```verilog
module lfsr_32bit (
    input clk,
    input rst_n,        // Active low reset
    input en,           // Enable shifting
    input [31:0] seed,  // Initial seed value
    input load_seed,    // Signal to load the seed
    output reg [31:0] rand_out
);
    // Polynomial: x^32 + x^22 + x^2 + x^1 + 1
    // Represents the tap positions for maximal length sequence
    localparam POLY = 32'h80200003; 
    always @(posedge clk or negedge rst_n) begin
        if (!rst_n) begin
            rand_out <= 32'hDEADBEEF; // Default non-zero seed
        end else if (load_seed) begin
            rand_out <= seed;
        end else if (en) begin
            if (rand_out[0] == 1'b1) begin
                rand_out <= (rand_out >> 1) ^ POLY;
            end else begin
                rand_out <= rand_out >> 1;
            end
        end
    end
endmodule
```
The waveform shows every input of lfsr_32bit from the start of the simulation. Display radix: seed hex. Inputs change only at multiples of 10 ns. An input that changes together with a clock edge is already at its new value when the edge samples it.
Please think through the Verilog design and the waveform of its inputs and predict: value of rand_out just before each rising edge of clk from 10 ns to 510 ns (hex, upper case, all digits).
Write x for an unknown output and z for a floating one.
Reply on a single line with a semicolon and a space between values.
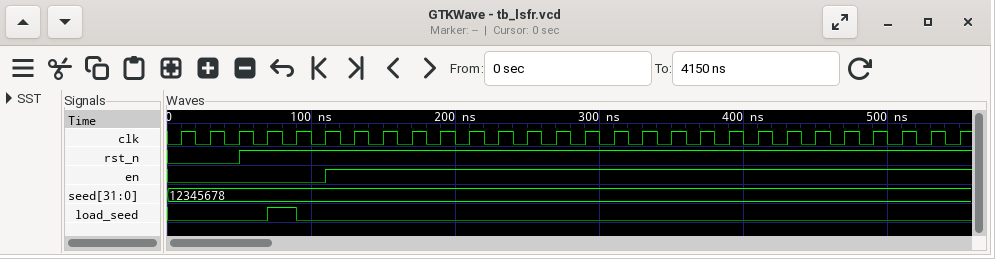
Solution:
DEADBEEF, DEADBEEF, DEADBEEF, DEADBEEF, 12345678, 12345678, 091A2B3C, 048D159E, 02468ACF, 81034564, 4081A2B2, 2040D159, 900068AF, C8203454, 64101A2A, 32080D15, 99240689, CCB20347, E67901A0, 733C80D0, 399E4068, 1CCF2034, 0E67901A, 0733C80D, 83B9E405, C1FCF201
